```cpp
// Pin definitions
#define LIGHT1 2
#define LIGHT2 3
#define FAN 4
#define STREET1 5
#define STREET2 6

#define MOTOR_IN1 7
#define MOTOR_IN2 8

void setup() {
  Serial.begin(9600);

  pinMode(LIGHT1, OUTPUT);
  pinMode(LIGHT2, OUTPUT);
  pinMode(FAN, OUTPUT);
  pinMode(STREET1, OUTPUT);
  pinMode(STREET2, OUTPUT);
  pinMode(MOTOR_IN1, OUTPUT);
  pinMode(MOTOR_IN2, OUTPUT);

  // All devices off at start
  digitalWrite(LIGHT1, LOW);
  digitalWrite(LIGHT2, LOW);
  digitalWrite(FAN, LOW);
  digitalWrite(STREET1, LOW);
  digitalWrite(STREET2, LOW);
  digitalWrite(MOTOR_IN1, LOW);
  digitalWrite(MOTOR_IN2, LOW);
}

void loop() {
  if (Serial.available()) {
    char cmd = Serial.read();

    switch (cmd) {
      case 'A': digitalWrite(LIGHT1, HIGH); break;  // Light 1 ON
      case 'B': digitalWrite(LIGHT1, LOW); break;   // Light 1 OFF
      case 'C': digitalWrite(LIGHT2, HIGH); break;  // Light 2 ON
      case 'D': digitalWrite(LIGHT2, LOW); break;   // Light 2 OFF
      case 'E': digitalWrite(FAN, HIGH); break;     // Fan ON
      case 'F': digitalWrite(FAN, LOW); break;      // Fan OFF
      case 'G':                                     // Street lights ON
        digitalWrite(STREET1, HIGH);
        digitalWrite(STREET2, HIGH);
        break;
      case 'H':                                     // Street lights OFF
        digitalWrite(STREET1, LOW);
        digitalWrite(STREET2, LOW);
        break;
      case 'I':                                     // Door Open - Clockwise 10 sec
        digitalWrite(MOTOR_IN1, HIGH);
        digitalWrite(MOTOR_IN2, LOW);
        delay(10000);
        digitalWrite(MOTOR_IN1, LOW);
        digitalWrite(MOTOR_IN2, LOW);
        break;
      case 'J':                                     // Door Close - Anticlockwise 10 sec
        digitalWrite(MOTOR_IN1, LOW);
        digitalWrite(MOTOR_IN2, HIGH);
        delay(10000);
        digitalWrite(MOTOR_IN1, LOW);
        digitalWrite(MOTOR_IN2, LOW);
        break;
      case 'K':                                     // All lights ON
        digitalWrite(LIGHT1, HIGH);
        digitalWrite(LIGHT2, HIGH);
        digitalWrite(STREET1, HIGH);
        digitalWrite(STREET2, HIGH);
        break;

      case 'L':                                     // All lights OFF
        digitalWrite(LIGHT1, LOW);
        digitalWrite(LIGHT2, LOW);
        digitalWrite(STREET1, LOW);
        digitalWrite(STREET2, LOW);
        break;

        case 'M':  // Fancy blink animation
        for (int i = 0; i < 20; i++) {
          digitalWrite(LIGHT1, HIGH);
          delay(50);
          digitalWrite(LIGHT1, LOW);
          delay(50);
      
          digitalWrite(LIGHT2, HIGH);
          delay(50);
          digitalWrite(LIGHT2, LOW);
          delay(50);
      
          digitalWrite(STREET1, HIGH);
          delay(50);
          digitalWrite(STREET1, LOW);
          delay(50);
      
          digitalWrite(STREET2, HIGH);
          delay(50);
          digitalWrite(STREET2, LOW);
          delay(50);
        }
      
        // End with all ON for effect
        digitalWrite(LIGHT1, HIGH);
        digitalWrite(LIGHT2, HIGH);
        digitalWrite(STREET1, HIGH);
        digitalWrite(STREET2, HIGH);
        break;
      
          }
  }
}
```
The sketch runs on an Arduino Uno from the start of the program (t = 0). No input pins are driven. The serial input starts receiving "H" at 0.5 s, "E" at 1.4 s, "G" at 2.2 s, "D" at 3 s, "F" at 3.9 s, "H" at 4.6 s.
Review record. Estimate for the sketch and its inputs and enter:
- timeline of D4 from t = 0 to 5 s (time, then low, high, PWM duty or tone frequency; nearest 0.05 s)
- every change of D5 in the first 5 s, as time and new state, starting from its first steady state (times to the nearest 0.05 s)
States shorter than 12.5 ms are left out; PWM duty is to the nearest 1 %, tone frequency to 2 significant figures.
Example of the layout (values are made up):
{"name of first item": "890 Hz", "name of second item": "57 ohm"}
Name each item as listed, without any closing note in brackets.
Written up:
{"timeline of D4 from t = 0 to 5 s": "0 s low; 1.4 s high; 3.9 s low", "every change of D5 in the first 5 s, as time and new state, starting from its first steady state": "0 s low; 2.2 s high; 4.6 s low"}
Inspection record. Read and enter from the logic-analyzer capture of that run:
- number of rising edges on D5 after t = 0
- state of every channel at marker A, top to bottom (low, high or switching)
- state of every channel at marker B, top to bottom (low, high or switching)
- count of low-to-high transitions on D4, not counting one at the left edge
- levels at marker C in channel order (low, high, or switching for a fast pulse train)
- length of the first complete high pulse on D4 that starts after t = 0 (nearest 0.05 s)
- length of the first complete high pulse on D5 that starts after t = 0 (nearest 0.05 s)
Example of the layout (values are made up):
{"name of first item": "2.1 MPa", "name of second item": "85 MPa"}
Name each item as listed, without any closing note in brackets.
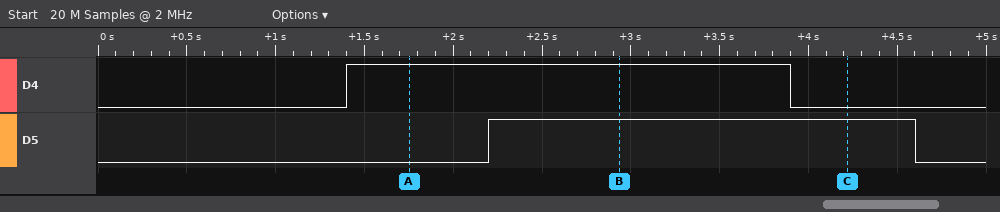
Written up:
{"number of rising edges on D5 after t = 0": "1", "state of every channel at marker A, top to bottom": "D4 high, D5 low", "state of every channel at marker B, top to bottom": "D4 high, D5 high", "count of low-to-high transitions on D4, not counting one at the left edge": "1", "levels at marker C in channel order": "D4 low, D5 high", "length of the first complete high pulse on D4 that starts after t = 0": "2.50 s", "length of the first complete high pulse on D5 that starts after t = 0": "2.40 s"}
